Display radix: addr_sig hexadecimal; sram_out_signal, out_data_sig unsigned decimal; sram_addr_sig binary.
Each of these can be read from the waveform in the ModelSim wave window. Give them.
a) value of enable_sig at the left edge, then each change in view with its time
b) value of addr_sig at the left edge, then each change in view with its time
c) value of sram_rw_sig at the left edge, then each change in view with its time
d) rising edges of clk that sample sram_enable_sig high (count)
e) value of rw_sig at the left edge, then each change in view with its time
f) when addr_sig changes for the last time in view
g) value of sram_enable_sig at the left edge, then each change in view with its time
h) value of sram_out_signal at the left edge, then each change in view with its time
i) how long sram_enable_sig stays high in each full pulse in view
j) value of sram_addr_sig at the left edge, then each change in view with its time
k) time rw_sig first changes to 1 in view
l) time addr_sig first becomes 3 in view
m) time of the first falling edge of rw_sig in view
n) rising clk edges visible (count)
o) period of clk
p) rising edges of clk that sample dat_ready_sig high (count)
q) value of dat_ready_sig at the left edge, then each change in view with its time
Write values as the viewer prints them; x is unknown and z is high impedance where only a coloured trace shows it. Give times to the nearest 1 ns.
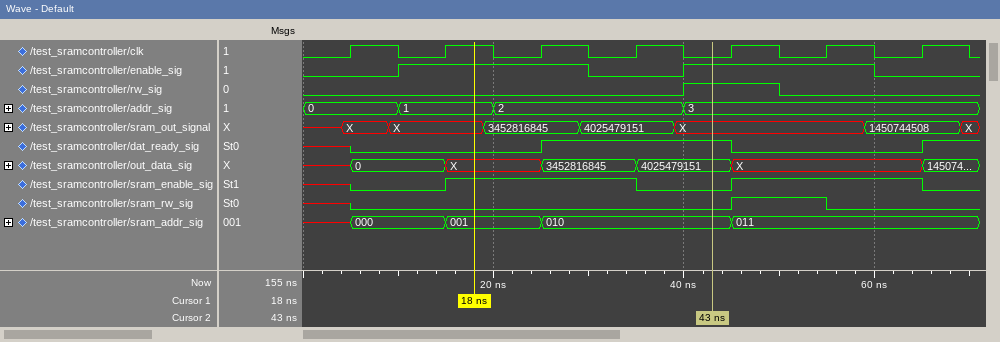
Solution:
0, 1 at 10 ns, 0 at 30 ns, 1 at 40 ns, 0 at 60 ns
0, 1 at 10 ns, 2 at 20 ns, 3 at 40 ns
x, 0 at 5 ns, 1 at 45 ns, 0 at 55 ns
4
0, 1 at 40 ns, 0 at 50 ns
40 ns
x, 0 at 5 ns, 1 at 15 ns, 0 at 35 ns, 1 at 45 ns, 0 at 65 ns
x, X at 4 ns, X at 9 ns, 3452816845 at 19 ns, 4025479151 at 29 ns, X at 39 ns, 1450744508 at 59 ns, X at 69 ns
20 ns, 20 ns
x, 000 at 5 ns, 001 at 15 ns, 010 at 25 ns, 011 at 45 ns
40 ns
40 ns
50 ns
7
10 ns
2
x, 0 at 5 ns, 1 at 25 ns, 0 at 45 ns, 1 at 65 ns
